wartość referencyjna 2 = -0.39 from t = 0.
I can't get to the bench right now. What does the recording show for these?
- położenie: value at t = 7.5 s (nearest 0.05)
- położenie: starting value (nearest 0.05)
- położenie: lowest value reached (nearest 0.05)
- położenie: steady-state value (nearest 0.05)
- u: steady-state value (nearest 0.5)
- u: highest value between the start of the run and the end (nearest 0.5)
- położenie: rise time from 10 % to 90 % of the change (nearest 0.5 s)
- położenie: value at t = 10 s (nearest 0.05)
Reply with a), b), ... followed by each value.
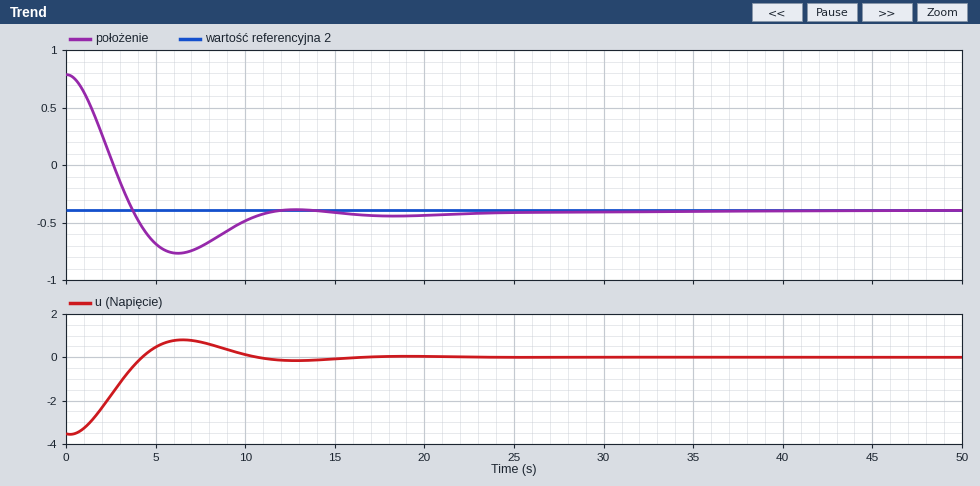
a) -0.70
b) 0.80
c) -0.75
d) -0.40
e) 0.0
f) 1.0
g) 2.5 s
h) -0.50
